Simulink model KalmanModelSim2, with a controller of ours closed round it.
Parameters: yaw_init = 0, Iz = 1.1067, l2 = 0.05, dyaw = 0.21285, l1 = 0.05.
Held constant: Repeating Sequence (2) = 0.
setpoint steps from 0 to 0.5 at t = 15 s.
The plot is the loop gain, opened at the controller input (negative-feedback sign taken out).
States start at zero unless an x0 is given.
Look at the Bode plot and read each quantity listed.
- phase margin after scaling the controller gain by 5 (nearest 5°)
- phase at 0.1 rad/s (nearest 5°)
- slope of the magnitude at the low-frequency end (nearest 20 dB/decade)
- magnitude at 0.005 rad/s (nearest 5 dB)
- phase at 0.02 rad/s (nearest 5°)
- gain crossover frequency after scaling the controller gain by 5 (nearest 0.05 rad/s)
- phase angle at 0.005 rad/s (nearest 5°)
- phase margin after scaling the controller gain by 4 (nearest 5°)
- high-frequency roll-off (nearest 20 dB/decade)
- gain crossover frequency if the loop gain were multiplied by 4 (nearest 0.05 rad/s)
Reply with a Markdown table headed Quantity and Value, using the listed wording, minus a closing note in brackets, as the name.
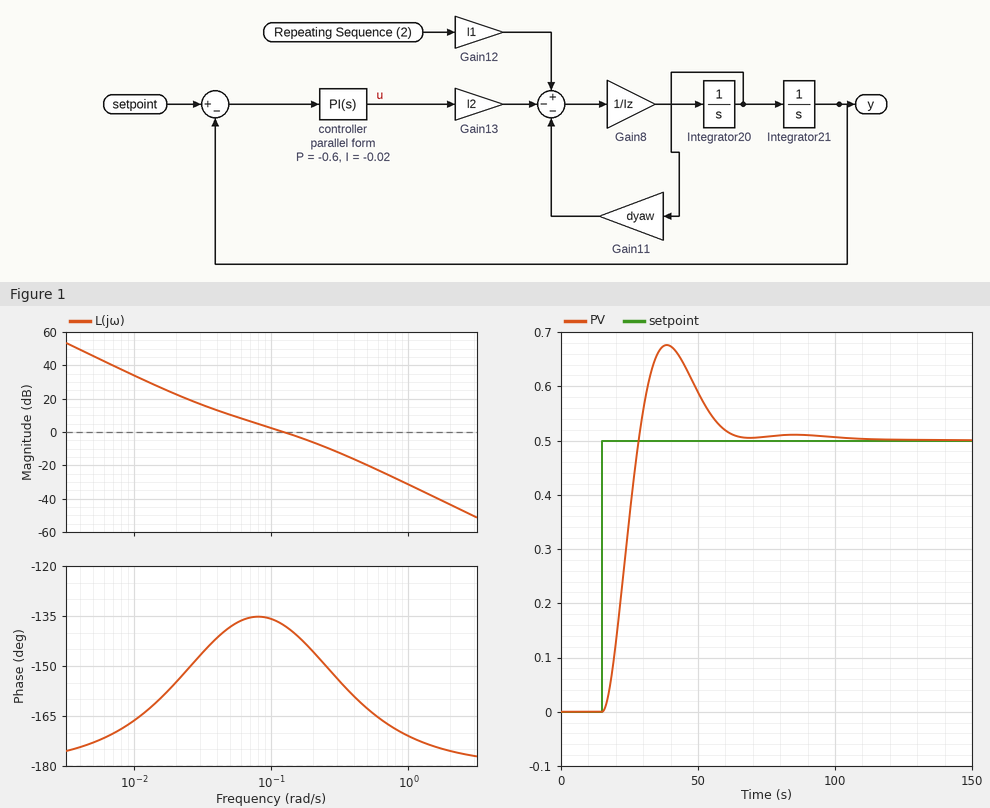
| Quantity | Value |
|---|---|
| phase margin after scaling the controller gain by 5 | 25° |
| phase at 0.1 rad/s | -135° |
| slope of the magnitude at the low-frequency end | -40 dB/decade |
| magnitude at 0.005 rad/s | 45 dB |
| phase at 0.02 rad/s | -155° |
| gain crossover frequency after scaling the controller gain by 5 | 0.35 rad/s |
| phase angle at 0.005 rad/s | -175° |
| phase margin after scaling the controller gain by 4 | 25° |
| high-frequency roll-off | -40 dB/decade |
| gain crossover frequency if the loop gain were multiplied by 4 | 0.30 rad/s |
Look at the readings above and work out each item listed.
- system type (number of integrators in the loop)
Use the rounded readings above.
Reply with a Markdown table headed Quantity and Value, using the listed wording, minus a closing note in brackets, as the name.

| Quantity | Value |
|---|---|
| system type | 2 |
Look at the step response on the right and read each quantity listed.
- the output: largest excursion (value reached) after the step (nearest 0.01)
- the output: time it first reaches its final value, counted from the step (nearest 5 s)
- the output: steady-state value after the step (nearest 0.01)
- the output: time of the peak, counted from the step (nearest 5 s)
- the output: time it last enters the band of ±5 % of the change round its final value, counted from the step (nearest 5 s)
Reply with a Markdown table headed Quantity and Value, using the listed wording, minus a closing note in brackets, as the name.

| Quantity | Value |
|---|---|
| the output: largest excursion (value reached) after the step | 0.68 |
| the output: time it first reaches its final value, counted from the step | 15 s |
| the output: steady-state value after the step | 0.50 |
| the output: time of the peak, counted from the step | 25 s |
| the output: time it last enters the band of ±5 % of the change round its final value, counted from the step | 45 s |
